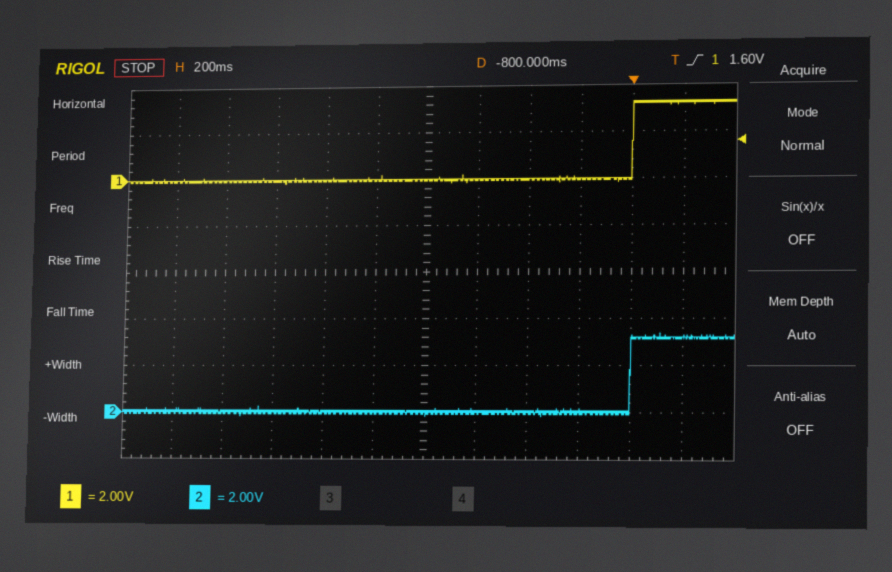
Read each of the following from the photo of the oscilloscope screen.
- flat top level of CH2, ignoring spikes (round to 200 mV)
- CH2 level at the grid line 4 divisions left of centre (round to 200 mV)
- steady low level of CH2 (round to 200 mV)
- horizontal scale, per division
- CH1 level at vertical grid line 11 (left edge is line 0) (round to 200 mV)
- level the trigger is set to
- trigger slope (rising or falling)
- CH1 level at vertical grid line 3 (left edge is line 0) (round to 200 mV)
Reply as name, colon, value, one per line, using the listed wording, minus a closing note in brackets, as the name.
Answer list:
flat top level of CH2, ignoring spikes: 3.2 V
CH2 level at the grid line 4 divisions left of centre: 0.0 V
steady low level of CH2: 0.0 V
horizontal scale, per division: 200 ms
CH1 level at vertical grid line 11 (left edge is line 0): 3.2 V
level the trigger is set to: 1.60 V
trigger slope: rising
CH1 level at vertical grid line 3 (left edge is line 0): 0.0 V
